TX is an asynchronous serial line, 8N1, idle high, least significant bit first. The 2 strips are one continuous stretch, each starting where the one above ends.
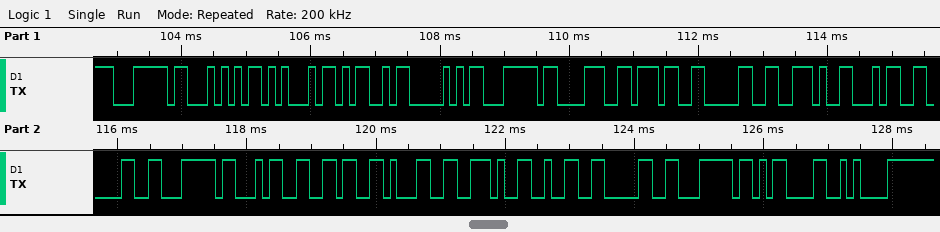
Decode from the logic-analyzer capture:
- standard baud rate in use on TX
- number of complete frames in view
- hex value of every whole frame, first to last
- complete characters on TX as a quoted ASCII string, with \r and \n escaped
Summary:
9600 baud
22
7C 54 45 4D 50 7C 38 37 30 2E 34 30 7C 34 36 31 2E 32 30 7C 0D 0A
"|TEMP|870.40|461.20|\r\n"
